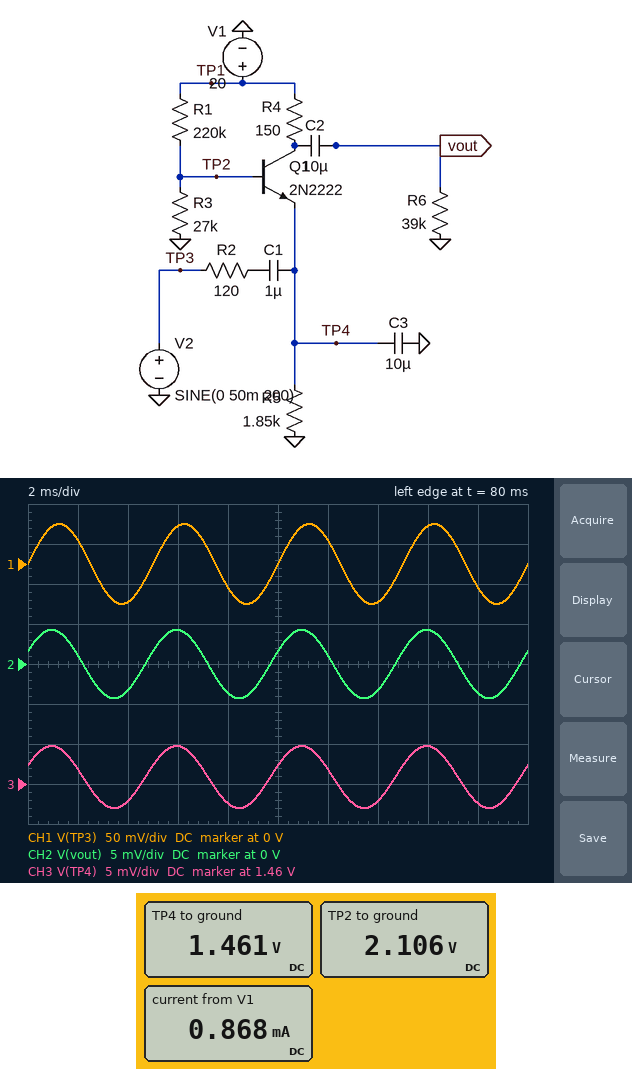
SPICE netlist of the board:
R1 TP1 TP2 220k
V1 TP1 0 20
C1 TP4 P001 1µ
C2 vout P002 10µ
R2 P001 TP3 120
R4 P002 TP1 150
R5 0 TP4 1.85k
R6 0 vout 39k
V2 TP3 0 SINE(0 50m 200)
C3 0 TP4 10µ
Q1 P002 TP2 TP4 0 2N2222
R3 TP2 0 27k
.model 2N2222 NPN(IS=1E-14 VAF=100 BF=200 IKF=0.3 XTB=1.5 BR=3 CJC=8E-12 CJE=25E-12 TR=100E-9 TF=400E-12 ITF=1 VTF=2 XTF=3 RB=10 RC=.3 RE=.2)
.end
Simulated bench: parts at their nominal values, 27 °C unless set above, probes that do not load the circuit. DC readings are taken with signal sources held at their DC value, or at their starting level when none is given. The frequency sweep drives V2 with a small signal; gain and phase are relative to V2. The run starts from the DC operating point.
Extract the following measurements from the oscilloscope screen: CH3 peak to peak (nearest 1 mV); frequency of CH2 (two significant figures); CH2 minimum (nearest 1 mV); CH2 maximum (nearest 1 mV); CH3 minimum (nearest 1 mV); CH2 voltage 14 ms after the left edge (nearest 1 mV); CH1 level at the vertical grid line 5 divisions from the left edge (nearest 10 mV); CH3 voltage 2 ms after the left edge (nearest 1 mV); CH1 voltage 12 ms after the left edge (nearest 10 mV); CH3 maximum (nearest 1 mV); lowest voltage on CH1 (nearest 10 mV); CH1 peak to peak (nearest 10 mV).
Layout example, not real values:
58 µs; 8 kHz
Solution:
8 mV; 200 Hz; -4 mV; 4 mV; 1.457 V; -3 mV; 0 V; 1.462 V; 30 mV; 1.465 V; -50 mV; 100 mV
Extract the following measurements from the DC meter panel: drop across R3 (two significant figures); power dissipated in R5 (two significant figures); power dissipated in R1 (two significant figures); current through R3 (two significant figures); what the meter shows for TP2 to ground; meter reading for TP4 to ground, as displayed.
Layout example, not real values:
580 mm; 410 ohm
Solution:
2.1 V; 1.2 mW; 1.5 mW; 78 µA; 2.106 V; 1.461 V
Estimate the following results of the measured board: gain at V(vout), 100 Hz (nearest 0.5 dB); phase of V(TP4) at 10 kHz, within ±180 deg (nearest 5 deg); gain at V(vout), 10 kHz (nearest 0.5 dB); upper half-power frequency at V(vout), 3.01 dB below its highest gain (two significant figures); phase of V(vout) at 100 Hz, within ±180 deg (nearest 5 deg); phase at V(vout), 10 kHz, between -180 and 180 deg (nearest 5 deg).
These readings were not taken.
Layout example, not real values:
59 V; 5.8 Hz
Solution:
-23.5 dB; -80 deg; -37.0 dB; 1.7 kHz; 45 deg; -80 deg
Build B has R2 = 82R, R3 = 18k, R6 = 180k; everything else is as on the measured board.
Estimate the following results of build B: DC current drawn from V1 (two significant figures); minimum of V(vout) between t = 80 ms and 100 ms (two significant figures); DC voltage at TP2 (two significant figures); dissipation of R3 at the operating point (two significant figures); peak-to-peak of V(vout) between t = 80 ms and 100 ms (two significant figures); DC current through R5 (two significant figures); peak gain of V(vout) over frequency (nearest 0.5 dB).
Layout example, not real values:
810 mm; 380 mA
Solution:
540 µA; -4.6 mV; 1.5 V; 120 µW; 9.1 mV; 460 µA; -20.0 dB
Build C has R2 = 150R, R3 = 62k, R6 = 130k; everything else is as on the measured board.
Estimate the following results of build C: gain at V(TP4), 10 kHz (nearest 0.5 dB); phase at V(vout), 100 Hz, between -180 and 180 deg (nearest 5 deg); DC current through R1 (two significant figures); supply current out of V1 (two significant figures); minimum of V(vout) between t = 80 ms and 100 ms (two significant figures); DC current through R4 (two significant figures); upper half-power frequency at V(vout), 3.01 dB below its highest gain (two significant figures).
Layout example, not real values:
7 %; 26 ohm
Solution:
-39.5 dB; 30 deg; 73 µA; 1.9 mA; -2.8 mV; 1.8 mA; 1.3 kHz
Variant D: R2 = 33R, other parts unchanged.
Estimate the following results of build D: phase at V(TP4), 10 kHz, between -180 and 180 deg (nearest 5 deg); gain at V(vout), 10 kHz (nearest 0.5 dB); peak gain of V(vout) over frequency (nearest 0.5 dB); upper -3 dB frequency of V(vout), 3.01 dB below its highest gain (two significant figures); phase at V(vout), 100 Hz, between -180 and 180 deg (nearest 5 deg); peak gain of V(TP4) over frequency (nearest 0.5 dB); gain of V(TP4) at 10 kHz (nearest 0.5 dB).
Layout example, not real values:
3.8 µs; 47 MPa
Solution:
-60 deg; -26.5 dB; -20.0 dB; 5.5 kHz; 50 deg; -21.0 dB; -27.5 dB
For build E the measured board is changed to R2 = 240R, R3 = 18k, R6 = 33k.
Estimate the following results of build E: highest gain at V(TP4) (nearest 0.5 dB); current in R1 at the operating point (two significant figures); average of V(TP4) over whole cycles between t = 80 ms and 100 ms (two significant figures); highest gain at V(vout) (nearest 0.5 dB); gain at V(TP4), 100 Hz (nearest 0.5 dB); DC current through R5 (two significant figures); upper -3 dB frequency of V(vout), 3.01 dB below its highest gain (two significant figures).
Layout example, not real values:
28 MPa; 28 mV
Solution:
-22.5 dB; 84 µA; 850 mV; -21.0 dB; -25.0 dB; 460 µA; 960 Hz
